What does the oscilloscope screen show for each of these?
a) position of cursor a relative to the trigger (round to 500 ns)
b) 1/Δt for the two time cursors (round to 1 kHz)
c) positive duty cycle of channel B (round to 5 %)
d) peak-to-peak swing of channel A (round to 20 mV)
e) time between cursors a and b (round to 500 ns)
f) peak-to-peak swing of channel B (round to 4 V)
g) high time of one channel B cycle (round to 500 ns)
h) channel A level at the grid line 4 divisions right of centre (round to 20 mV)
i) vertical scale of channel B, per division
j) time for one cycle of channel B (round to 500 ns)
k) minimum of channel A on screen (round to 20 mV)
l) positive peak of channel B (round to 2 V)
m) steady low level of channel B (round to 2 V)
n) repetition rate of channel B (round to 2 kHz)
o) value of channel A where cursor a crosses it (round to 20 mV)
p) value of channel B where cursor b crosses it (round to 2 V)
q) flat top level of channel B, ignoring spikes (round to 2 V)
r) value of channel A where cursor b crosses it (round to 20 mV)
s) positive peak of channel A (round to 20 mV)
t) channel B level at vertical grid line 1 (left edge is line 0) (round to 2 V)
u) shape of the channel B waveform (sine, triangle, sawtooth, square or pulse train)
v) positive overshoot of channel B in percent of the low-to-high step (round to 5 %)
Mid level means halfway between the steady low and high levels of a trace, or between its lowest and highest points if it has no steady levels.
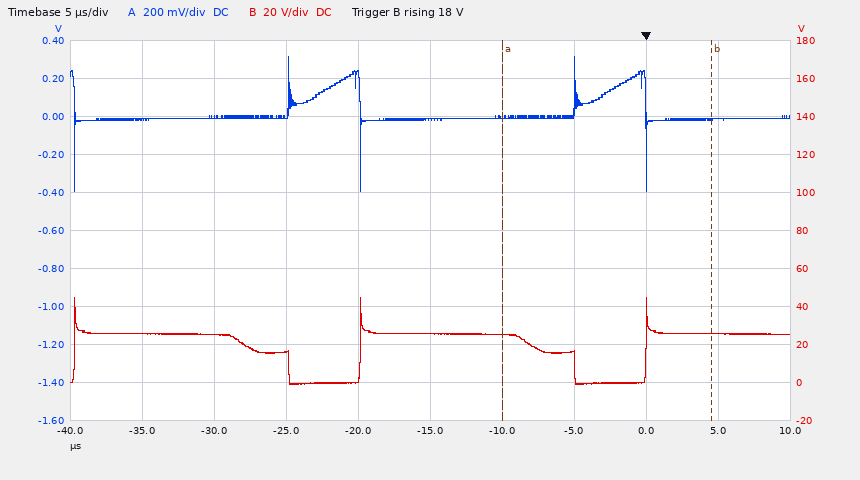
-10.0 µs
69 kHz
75 %
720 mV
14.5 µs
44 V
15.0 µs
-20 mV
20 V
20.0 µs
-400 mV
44 V
0 V
50 kHz
0 mV
26 V
26 V
-20 mV
320 mV
26 V
pulse train
75 %
